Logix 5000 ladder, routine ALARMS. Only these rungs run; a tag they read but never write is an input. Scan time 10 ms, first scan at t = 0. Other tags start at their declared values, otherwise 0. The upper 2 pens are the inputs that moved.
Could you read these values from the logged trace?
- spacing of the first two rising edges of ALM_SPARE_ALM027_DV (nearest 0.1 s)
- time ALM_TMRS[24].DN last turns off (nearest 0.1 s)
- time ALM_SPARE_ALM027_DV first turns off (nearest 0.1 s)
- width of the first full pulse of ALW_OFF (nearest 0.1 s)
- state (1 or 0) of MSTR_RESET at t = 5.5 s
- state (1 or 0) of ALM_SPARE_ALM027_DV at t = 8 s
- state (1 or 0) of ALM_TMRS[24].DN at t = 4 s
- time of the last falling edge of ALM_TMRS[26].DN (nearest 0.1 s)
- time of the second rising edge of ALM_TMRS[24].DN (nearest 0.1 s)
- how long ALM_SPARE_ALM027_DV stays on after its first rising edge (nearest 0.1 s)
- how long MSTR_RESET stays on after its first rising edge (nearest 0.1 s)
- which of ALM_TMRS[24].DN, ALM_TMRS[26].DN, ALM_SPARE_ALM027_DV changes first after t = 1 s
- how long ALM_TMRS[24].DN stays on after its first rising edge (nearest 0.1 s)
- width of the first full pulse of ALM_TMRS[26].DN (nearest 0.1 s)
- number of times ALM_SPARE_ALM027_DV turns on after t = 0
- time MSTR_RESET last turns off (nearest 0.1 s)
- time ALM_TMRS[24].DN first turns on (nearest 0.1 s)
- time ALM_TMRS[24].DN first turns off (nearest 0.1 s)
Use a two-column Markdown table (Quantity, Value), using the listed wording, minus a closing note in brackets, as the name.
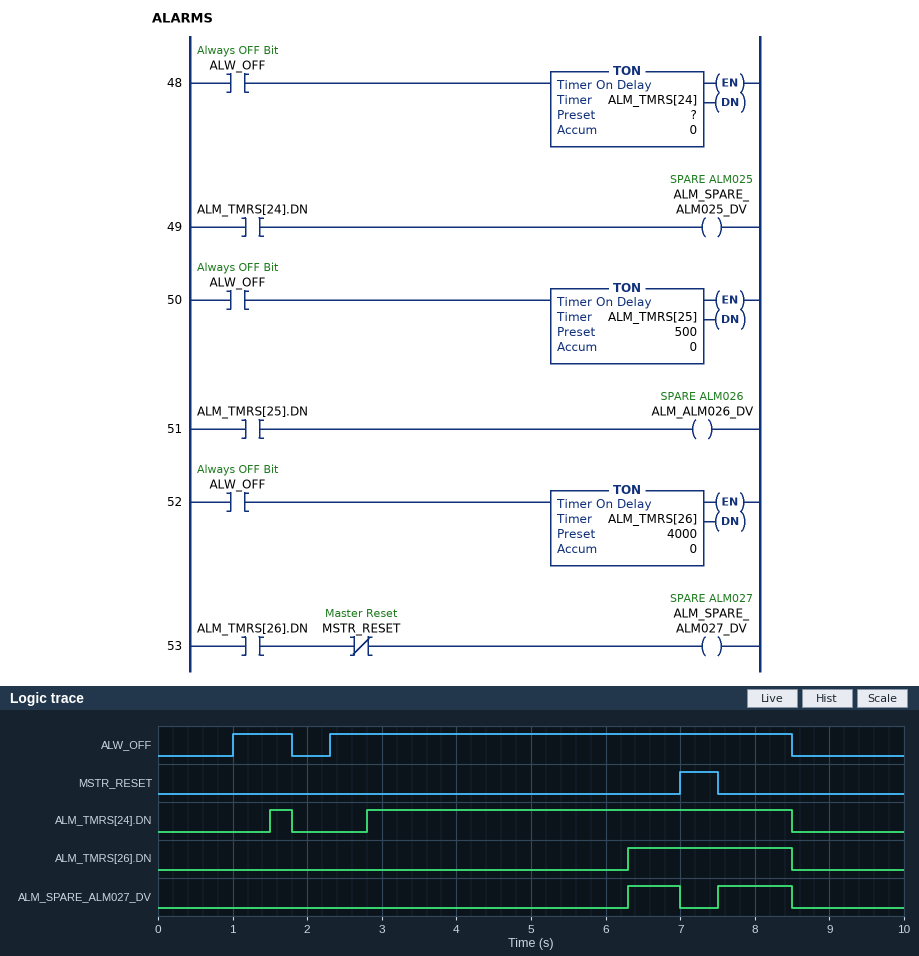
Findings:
| Quantity | Value |
|---|---|
| spacing of the first two rising edges of ALM_SPARE_ALM027_DV | 1.2 s |
| time ALM_TMRS[24].DN last turns off | 8.5 s |
| time ALM_SPARE_ALM027_DV first turns off | 7.0 s |
| width of the first full pulse of ALW_OFF | 0.8 s |
| state (1 or 0) of MSTR_RESET at t = 5.5 s | 0 |
| state (1 or 0) of ALM_SPARE_ALM027_DV at t = 8 s | 1 |
| state (1 or 0) of ALM_TMRS[24].DN at t = 4 s | 1 |
| time of the last falling edge of ALM_TMRS[26].DN | 8.5 s |
| time of the second rising edge of ALM_TMRS[24].DN | 2.8 s |
| how long ALM_SPARE_ALM027_DV stays on after its first rising edge | 0.7 s |
| how long MSTR_RESET stays on after its first rising edge | 0.5 s |
| which of ALM_TMRS[24].DN, ALM_TMRS[26].DN, ALM_SPARE_ALM027_DV changes first after t = 1 s | ALM_TMRS[24].DN |
| how long ALM_TMRS[24].DN stays on after its first rising edge | 0.3 s |
| width of the first full pulse of ALM_TMRS[26].DN | 2.2 s |
| number of times ALM_SPARE_ALM027_DV turns on after t = 0 | 2 |
| time MSTR_RESET last turns off | 7.5 s |
| time ALM_TMRS[24].DN first turns on | 1.5 s |
| time ALM_TMRS[24].DN first turns off | 1.8 s |
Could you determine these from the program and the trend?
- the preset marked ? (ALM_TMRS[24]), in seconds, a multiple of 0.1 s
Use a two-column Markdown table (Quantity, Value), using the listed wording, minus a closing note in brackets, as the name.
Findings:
| Quantity | Value |
|---|---|
| the preset marked ? (ALM_TMRS[24]), in seconds, a multiple of 0.1 s | 0.5 s |
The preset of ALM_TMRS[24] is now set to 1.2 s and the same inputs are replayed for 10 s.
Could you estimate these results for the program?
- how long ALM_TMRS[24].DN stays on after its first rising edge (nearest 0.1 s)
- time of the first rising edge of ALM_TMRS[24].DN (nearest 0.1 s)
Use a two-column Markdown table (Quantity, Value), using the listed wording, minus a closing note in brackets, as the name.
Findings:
| Quantity | Value |
|---|---|
| how long ALM_TMRS[24].DN stays on after its first rising edge | 5.0 s |
| time of the first rising edge of ALM_TMRS[24].DN | 3.5 s |
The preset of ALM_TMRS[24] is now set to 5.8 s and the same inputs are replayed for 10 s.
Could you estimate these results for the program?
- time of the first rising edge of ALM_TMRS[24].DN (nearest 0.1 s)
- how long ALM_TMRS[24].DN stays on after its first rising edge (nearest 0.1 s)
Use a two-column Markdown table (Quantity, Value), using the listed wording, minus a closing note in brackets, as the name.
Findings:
| Quantity | Value |
|---|---|
| time of the first rising edge of ALM_TMRS[24].DN | 8.1 s |
| how long ALM_TMRS[24].DN stays on after its first rising edge | 0.4 s |
